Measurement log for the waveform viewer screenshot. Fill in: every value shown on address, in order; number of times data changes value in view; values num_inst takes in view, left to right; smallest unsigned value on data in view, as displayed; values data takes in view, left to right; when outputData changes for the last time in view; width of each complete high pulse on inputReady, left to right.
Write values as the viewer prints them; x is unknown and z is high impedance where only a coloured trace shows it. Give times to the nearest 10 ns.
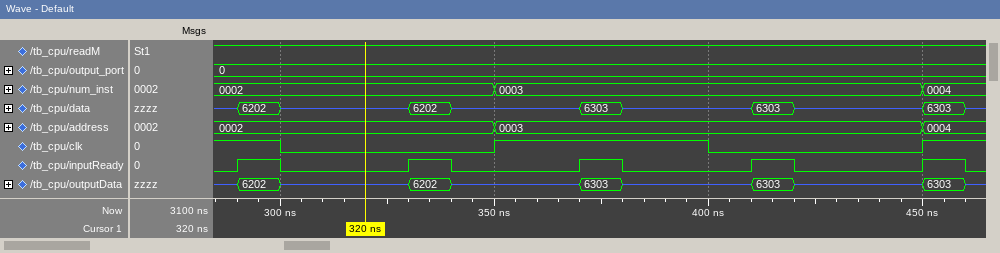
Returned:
0002, 0003, 0004
10
0002, 0003, 0004
6202
z, 6202, z, 6202, z, 6303, z, 6303, z, 6303, z
460 ns
10 ns, 10 ns, 10 ns, 10 ns, 10 ns
